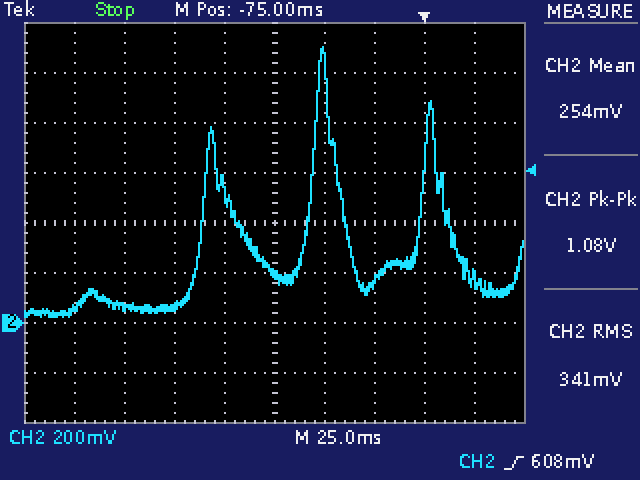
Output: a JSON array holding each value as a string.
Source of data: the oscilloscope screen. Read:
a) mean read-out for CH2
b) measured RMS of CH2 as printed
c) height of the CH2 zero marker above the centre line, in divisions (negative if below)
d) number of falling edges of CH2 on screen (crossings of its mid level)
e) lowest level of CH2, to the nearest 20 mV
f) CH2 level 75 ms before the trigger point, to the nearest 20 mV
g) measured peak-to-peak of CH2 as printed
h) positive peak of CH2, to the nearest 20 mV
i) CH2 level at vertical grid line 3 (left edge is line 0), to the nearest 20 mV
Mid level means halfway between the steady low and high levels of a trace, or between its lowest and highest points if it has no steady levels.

["254 mV", "341 mV", "-2.0 div", "3", "20 mV", "200 mV", "1.08 V", "1.10 V", "60 mV"]
